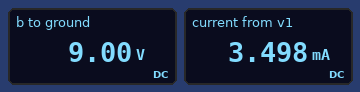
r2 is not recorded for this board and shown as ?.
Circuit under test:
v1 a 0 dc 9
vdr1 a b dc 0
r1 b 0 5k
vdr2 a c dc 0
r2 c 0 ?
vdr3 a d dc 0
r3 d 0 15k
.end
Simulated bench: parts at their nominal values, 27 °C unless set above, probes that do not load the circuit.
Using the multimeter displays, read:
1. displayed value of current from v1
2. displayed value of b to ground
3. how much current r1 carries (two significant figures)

3.498 mA
9.00 V
1.8 mA
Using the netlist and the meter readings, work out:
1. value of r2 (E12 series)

8.2 kΩ
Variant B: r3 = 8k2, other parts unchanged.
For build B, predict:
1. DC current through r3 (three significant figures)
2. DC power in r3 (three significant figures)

1.10 mA
9.88 mW
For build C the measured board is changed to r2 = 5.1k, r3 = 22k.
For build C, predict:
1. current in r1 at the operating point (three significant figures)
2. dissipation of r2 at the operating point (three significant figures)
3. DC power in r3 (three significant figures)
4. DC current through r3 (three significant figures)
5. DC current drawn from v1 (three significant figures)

1.80 mA
15.9 mW
3.68 mW
409 µA
3.97 mA
